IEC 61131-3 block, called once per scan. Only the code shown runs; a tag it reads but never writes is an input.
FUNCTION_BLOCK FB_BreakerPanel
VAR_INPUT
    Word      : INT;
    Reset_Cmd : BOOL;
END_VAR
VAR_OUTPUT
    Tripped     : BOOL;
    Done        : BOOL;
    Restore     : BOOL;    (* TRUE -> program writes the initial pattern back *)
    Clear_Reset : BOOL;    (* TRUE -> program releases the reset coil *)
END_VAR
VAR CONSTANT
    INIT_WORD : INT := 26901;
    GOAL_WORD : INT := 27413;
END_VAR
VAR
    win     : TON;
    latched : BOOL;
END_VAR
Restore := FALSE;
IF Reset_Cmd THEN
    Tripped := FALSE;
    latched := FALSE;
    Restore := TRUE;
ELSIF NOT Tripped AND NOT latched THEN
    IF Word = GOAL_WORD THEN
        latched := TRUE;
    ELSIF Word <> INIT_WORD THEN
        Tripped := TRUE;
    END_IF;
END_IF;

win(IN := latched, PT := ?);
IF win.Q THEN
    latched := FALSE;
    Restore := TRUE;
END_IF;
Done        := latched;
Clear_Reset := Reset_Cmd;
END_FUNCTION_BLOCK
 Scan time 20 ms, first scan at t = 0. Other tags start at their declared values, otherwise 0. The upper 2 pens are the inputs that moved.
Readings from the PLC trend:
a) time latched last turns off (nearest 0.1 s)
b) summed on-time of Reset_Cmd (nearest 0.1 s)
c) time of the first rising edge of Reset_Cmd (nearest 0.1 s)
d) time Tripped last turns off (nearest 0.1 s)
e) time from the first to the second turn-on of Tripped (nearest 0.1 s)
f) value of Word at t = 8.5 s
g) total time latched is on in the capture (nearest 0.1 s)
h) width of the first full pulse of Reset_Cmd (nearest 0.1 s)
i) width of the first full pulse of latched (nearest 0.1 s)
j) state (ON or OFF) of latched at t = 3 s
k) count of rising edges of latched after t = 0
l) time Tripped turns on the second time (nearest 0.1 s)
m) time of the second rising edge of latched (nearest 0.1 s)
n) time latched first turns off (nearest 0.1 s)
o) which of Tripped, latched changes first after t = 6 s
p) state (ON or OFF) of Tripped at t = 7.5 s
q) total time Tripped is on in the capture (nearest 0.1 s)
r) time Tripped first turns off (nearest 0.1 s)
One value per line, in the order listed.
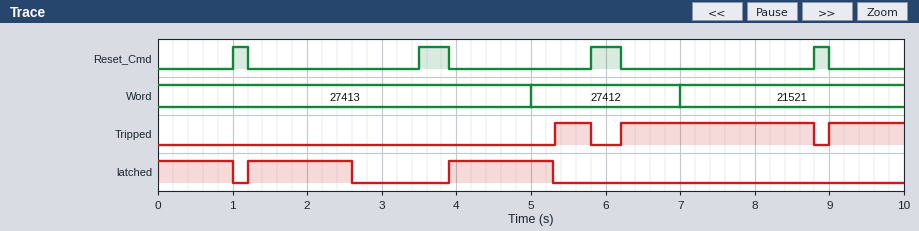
5.3 s
1.2 s
1.0 s
8.8 s
0.9 s
21521
3.8 s
0.2 s
1.4 s
OFF
2
6.2 s
3.9 s
1.0 s
Tripped
ON
4.1 s
5.8 s
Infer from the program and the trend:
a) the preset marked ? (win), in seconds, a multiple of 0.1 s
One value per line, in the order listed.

1.4 s
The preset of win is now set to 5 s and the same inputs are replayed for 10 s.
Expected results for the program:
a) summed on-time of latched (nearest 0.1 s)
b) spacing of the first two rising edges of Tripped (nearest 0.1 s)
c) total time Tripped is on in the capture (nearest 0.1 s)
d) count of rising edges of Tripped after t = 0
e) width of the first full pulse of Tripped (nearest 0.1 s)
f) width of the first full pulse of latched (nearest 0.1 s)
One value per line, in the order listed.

5.2 s
2.8 s
3.6 s
2
2.6 s
2.3 s
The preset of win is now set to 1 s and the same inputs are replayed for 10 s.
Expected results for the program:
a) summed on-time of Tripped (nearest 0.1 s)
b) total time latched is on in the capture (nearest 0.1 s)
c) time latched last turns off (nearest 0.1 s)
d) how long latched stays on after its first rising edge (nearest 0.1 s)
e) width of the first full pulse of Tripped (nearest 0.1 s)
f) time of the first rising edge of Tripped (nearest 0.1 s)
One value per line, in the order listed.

4.4 s
3.0 s
4.9 s
1.0 s
0.8 s
5.0 s
